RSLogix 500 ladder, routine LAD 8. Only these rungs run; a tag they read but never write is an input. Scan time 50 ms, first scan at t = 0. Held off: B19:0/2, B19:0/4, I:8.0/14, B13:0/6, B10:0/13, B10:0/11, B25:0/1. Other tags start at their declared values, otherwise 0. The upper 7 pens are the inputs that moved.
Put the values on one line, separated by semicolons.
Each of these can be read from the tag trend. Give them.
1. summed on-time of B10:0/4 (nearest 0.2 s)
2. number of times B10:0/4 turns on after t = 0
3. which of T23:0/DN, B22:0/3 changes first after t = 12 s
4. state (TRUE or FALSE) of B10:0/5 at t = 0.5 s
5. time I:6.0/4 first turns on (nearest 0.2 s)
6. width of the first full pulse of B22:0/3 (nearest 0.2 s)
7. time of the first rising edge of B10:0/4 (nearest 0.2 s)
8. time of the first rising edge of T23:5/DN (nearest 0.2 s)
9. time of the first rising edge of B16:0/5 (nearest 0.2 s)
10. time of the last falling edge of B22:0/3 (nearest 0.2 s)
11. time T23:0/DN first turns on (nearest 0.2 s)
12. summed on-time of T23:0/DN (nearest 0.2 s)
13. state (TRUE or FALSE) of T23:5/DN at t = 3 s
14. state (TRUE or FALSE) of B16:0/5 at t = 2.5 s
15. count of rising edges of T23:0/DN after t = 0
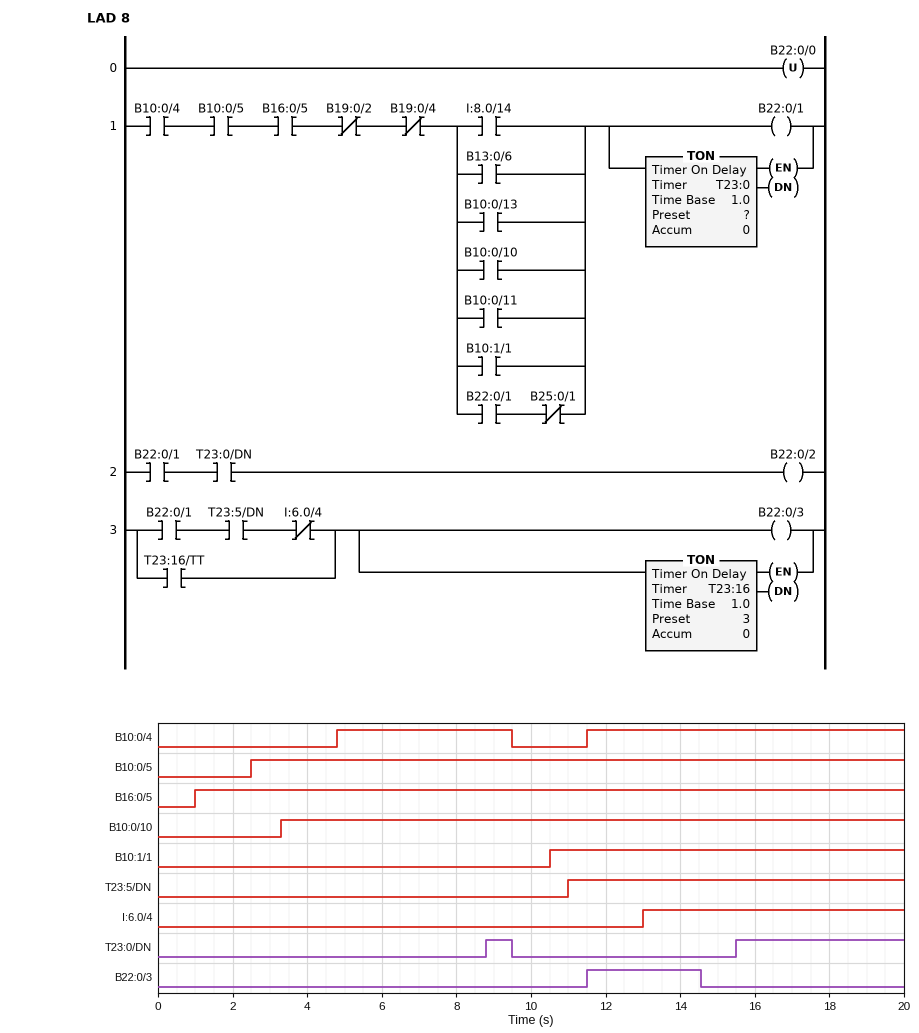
13.2 s; 2; B22:0/3; FALSE; 13.0 s; 3.0 s; 4.8 s; 11.0 s; 1.0 s; 14.6 s; 8.8 s; 5.2 s; FALSE; TRUE; 2
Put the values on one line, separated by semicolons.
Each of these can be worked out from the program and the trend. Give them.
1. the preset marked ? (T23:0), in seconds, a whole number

4 s
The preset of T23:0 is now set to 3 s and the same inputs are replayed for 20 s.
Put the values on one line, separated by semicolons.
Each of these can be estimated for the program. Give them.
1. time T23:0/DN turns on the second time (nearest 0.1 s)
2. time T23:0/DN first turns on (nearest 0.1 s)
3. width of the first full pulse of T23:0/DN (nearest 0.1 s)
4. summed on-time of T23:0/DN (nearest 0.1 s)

14.5 s; 7.8 s; 1.7 s; 7.2 s
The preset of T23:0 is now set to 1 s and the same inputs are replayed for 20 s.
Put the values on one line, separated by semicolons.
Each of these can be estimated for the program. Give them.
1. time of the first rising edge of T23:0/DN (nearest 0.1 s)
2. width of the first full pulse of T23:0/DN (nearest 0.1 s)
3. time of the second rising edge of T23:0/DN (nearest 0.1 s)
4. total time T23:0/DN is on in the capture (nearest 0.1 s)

5.8 s; 3.7 s; 12.5 s; 11.2 s
